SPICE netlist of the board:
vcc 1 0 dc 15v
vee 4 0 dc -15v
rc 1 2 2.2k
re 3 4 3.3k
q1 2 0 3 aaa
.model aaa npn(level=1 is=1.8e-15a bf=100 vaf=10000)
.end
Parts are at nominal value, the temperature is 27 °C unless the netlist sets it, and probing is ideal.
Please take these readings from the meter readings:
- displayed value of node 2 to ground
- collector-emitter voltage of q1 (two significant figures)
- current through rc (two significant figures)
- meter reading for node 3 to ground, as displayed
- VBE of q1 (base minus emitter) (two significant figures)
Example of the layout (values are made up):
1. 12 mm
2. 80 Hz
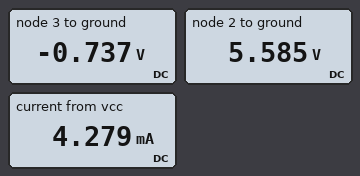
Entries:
1. 5.585 V
2. 6.3 V
3. 4.3 mA
4. -0.737 V
5. 740 mV
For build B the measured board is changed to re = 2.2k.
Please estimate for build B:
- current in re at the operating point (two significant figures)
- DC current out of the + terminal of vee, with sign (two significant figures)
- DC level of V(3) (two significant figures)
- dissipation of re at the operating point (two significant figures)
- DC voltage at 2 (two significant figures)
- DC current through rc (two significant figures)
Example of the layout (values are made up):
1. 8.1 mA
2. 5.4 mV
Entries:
1. 6.5 mA
2. -6.5 mA
3. -750 mV
4. 92 mW
5. 890 mV
6. 6.4 mA
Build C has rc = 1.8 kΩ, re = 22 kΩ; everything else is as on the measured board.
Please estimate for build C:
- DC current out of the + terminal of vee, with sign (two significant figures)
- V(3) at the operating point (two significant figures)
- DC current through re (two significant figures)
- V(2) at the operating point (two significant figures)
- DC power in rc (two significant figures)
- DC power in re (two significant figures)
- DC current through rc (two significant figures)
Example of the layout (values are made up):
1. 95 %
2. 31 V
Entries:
1. -650 µA
2. -690 mV
3. 650 µA
4. 14 V
5. 750 µW
6. 9.3 mW
7. 640 µA
